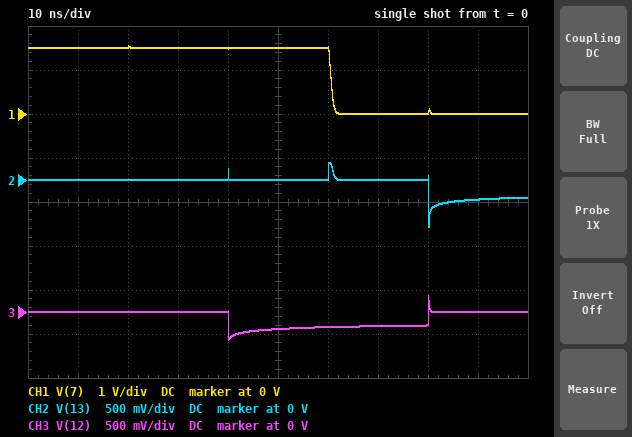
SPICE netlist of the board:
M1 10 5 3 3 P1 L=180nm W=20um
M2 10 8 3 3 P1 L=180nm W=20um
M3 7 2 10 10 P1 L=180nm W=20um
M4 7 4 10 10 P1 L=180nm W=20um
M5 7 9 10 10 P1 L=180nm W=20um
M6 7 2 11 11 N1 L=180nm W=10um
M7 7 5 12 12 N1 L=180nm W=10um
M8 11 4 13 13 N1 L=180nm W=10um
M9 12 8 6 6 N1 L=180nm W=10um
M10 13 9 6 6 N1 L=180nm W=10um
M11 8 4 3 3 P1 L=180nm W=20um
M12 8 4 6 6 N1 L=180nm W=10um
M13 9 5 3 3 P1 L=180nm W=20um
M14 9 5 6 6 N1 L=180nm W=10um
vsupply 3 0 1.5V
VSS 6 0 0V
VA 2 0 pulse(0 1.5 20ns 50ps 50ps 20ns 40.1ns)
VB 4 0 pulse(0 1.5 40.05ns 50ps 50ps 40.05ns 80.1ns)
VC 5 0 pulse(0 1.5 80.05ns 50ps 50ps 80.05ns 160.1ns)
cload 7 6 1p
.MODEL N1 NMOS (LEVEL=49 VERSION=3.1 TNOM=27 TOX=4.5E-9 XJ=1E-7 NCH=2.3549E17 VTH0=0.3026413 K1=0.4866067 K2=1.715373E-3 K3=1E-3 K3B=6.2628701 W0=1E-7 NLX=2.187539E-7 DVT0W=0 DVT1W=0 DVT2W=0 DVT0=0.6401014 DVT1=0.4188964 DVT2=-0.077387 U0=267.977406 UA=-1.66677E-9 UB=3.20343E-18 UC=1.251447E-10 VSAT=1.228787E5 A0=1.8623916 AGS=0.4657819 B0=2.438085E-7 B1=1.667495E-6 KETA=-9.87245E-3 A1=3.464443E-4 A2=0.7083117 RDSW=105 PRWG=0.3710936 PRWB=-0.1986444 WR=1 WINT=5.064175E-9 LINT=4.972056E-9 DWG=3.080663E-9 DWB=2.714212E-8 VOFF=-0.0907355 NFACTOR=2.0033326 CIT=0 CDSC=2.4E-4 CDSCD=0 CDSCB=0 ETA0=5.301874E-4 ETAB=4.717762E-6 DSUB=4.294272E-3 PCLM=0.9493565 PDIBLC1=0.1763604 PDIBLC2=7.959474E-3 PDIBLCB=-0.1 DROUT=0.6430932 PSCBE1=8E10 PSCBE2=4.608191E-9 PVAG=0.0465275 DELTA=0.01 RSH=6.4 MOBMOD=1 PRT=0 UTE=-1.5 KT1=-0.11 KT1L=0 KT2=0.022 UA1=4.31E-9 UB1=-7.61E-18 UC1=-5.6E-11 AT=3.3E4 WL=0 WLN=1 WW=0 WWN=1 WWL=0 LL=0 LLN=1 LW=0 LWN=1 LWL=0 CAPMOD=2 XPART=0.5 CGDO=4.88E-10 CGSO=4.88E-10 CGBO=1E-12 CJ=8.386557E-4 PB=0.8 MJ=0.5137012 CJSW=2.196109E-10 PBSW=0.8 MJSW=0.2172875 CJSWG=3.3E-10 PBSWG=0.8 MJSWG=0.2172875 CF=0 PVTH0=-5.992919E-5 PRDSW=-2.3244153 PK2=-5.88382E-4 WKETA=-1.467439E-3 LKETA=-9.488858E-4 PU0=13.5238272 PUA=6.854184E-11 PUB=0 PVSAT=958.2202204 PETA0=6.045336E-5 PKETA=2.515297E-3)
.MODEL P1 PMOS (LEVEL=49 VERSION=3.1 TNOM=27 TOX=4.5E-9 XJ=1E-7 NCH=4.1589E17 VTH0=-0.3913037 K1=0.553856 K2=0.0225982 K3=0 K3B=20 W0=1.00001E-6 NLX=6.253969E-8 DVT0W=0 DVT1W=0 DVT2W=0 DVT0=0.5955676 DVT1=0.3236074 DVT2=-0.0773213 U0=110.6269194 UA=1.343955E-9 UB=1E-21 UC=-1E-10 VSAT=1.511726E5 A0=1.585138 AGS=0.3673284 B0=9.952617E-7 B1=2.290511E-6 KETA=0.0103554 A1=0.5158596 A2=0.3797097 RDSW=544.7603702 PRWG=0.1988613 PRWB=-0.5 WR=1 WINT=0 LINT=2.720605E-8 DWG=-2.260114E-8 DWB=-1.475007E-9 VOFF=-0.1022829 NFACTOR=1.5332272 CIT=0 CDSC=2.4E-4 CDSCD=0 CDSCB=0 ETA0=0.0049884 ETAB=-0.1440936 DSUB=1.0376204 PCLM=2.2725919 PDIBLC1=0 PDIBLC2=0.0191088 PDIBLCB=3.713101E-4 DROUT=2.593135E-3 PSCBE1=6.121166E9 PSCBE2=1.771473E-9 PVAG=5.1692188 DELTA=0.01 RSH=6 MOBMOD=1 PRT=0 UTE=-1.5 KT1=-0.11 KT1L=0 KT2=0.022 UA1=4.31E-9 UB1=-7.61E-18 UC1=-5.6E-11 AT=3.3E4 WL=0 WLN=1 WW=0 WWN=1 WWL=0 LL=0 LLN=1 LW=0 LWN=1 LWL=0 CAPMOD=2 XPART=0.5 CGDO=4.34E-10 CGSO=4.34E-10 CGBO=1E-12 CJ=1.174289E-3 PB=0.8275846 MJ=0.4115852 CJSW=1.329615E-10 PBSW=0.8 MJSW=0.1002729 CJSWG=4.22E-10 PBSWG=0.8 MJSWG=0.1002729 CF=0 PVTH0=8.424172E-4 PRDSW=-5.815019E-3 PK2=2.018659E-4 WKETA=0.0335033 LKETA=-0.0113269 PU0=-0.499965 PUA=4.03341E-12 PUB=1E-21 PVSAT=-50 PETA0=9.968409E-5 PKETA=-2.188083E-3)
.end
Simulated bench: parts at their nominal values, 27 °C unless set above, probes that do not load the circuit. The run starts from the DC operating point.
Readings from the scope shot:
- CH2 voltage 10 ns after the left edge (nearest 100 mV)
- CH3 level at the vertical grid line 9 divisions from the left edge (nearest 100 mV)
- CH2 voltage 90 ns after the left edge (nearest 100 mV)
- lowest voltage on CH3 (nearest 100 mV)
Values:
0 V
0 V
-200 mV
-300 mV
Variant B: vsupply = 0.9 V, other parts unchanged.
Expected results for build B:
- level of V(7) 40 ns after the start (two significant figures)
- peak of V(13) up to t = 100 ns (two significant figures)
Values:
900 mV
420 mV
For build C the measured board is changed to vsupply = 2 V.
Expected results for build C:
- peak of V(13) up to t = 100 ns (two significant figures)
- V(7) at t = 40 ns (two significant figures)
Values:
170 mV
2.0 V
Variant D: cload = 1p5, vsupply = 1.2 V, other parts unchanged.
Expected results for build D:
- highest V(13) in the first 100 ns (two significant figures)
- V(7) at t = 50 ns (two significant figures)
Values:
250 mV
1.2 V
